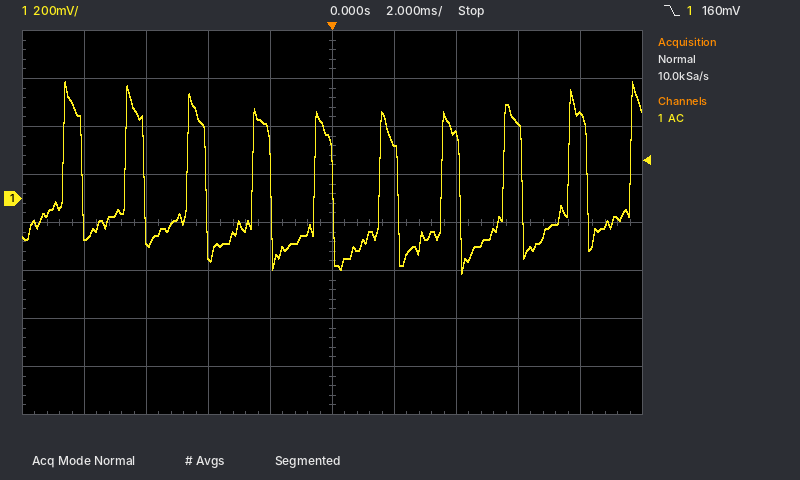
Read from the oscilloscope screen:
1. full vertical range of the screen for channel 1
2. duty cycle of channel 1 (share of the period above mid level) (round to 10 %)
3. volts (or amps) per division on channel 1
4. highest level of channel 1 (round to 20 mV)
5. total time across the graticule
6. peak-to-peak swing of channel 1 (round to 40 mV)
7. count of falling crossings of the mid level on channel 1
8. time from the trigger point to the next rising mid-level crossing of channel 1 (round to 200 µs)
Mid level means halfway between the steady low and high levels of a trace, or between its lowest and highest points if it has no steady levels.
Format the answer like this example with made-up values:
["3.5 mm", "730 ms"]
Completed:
["1.6 V", "30 %", "200 mV", "480 mV", "20 ms", "800 mV", "9", "1.6 ms"]
